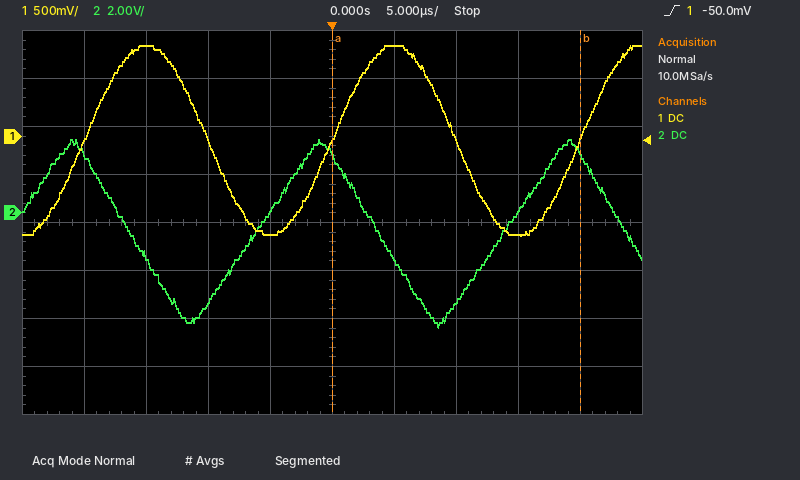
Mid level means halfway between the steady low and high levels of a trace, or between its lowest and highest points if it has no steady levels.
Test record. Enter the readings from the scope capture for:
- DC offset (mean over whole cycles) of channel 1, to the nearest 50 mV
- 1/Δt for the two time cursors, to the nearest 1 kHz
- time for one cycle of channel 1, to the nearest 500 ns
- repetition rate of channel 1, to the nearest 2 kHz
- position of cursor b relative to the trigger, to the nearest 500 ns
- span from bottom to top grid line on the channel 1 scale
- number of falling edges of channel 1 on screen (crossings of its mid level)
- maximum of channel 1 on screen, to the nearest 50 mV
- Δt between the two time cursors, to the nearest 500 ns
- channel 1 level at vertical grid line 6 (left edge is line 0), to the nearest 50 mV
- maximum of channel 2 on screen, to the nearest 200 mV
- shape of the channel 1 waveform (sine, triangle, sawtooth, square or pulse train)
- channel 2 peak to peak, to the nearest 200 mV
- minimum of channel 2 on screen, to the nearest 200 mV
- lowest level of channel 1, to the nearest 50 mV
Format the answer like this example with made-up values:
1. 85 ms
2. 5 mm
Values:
1. -50 mV
2. 50 kHz
3. 20.0 µs
4. 50 kHz
5. +20.0 µs
6. 4 V
7. 2
8. 950 mV
9. 20.0 µs
10. 950 mV
11. 3.0 V
12. sine
13. 7.8 V
14. -4.8 V
15. -1.05 V
